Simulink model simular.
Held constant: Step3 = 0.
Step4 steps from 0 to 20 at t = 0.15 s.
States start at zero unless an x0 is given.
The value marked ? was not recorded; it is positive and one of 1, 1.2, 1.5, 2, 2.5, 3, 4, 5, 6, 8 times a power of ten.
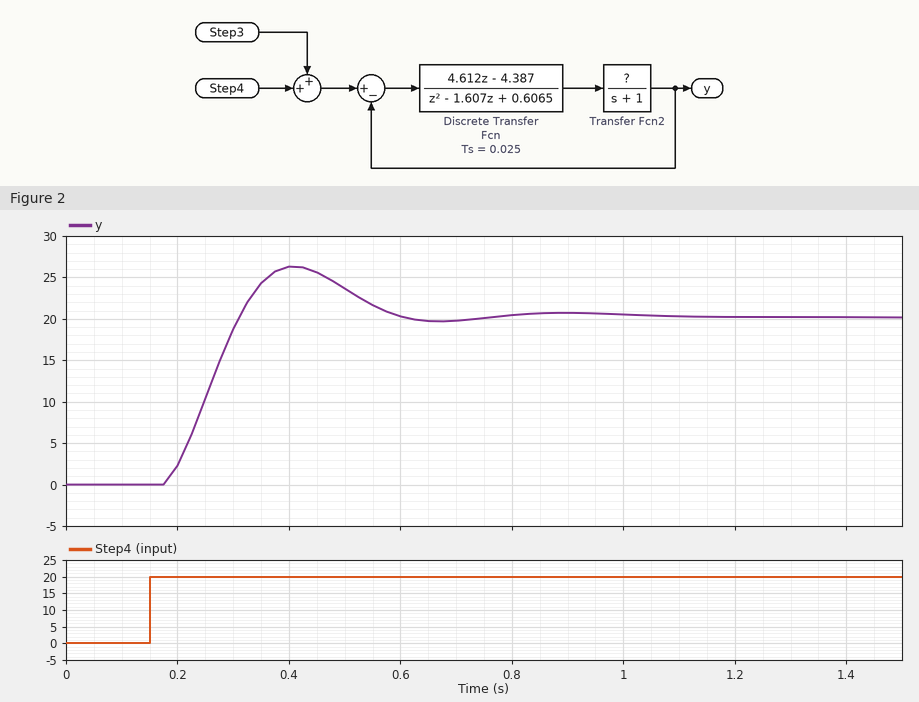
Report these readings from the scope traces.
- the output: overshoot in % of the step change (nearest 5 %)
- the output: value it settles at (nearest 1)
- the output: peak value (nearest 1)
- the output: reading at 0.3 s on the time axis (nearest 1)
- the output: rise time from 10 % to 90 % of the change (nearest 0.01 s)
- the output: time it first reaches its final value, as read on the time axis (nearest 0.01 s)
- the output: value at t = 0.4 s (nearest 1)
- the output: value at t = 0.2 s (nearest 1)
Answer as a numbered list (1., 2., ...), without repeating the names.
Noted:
1. 30 %
2. 20
3. 26
4. 19
5. 0.10 s
6. 0.31 s
7. 26
8. 2
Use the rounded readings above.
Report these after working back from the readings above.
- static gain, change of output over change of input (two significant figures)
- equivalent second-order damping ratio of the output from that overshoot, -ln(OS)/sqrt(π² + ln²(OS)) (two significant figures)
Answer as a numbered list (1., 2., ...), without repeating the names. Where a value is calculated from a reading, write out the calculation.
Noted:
1. (20 - 0) / (20 - 0) = 1.0
2. ln(0.3) = -1.204; 1.204 / sqrt(9.870 + 1.450) = 0.36
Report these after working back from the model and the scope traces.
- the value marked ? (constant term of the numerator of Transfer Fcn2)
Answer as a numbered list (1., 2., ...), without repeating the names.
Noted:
1. 1
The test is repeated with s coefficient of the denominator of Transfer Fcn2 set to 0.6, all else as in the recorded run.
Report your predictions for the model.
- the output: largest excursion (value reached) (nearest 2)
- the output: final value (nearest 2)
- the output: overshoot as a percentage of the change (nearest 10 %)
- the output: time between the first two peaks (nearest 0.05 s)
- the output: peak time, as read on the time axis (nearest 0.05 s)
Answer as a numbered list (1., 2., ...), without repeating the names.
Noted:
1. 30
2. 20
3. 50 %
4. 0.35 s
5. 0.35 s
